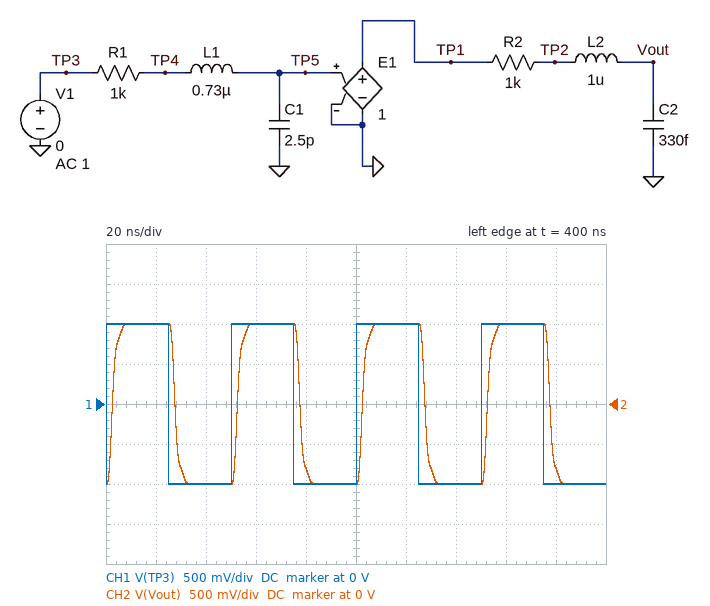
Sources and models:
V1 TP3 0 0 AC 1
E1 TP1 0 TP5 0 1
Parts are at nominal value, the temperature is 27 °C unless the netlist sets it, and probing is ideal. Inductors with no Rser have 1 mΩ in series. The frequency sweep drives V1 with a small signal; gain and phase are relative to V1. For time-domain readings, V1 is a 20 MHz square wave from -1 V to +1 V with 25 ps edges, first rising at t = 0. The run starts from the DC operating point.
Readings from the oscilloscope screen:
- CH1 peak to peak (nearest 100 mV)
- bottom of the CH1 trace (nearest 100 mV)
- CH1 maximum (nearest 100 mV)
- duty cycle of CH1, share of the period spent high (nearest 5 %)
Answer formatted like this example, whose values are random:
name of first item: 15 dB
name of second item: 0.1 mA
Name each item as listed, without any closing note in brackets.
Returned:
CH1 peak to peak: 2.0 V
bottom of the CH1 trace: -1.0 V
CH1 maximum: 1.0 V
duty cycle of CH1, share of the period spent high: 50 %
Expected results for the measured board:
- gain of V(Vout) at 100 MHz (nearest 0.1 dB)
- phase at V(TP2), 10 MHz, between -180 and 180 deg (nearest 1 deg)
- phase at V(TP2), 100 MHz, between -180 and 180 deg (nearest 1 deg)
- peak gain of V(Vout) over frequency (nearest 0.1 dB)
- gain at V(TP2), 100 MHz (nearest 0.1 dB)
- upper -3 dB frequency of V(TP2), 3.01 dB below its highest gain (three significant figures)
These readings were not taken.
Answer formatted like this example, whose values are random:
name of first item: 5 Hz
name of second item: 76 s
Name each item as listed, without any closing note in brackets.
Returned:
gain of V(Vout) at 100 MHz: -3.1 dB
phase at V(TP2), 10 MHz, between -180 and 180 deg: -10 deg
phase at V(TP2), 100 MHz, between -180 and 180 deg: -93 deg
peak gain of V(Vout) over frequency: 0 dB
gain at V(TP2), 100 MHz: -4.3 dB
upper -3 dB frequency of V(TP2), 3.01 dB below its highest gain: 82.3 MHz
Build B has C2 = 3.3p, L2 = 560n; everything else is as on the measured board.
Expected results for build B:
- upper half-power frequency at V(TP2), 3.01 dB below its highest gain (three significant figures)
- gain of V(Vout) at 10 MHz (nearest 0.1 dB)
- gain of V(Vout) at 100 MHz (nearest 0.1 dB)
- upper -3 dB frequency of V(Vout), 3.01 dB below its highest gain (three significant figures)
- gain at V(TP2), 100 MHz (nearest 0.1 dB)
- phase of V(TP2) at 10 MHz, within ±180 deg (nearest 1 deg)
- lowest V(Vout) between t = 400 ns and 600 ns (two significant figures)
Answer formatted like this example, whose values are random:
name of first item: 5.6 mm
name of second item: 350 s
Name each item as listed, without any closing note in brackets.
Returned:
upper half-power frequency at V(TP2), 3.01 dB below its highest gain: 37.2 MHz
gain of V(Vout) at 10 MHz: -0.2 dB
gain of V(Vout) at 100 MHz: -10.5 dB
upper -3 dB frequency of V(Vout), 3.01 dB below its highest gain: 45.7 MHz
gain at V(TP2), 100 MHz: -21.8 dB
phase of V(TP2) at 10 MHz, within ±180 deg: -21 deg
lowest V(Vout) between t = 400 ns and 600 ns: -1.0 V
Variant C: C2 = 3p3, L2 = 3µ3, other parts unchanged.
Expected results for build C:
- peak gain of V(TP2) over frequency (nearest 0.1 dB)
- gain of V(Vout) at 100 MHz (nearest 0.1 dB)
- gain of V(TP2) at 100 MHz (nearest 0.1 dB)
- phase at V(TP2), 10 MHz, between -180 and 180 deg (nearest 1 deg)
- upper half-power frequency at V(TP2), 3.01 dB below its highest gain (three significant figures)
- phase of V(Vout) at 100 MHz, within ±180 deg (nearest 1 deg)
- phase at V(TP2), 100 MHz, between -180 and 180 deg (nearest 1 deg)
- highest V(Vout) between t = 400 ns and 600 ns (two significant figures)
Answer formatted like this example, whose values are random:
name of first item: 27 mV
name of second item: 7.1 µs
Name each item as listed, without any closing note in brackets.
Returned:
peak gain of V(TP2) over frequency: 0 dB
gain of V(Vout) at 100 MHz: -15.9 dB
gain of V(TP2) at 100 MHz: -5.5 dB
phase at V(TP2), 10 MHz, between -180 and 180 deg: -21 deg
upper half-power frequency at V(TP2), 3.01 dB below its highest gain: 28.6 MHz
phase of V(Vout) at 100 MHz, within ±180 deg: 132 deg
phase at V(TP2), 100 MHz, between -180 and 180 deg: -48 deg
highest V(Vout) between t = 400 ns and 600 ns: 1.3 V
